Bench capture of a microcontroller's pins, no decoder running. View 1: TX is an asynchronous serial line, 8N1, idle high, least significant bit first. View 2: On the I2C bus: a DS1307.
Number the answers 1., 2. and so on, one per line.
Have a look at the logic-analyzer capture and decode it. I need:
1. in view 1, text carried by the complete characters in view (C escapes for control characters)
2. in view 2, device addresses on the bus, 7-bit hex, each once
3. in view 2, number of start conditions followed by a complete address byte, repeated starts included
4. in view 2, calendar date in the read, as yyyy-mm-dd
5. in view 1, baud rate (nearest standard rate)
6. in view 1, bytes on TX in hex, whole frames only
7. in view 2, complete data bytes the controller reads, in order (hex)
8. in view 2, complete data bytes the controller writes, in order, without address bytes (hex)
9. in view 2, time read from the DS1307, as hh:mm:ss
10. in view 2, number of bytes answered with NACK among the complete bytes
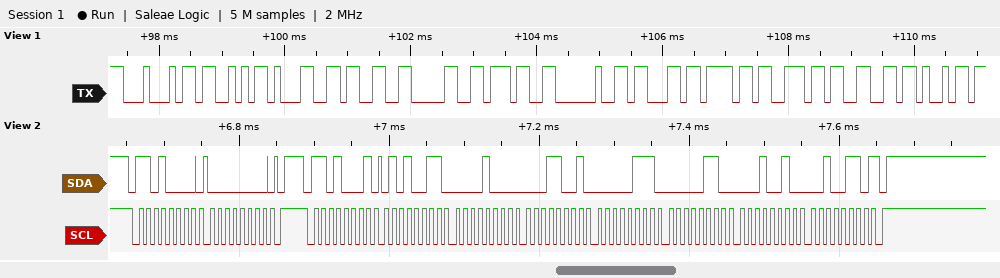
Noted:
1. "DS1307 confi"
2. 0x68
3. 2
4. 2026-12-06
5. 9600 baud
6. 44 53 31 33 30 37 20 63 6F 6E 66 69
7. 53 08 19 07 06 12 26
8. 00
9. 19:08:53
10. 1
